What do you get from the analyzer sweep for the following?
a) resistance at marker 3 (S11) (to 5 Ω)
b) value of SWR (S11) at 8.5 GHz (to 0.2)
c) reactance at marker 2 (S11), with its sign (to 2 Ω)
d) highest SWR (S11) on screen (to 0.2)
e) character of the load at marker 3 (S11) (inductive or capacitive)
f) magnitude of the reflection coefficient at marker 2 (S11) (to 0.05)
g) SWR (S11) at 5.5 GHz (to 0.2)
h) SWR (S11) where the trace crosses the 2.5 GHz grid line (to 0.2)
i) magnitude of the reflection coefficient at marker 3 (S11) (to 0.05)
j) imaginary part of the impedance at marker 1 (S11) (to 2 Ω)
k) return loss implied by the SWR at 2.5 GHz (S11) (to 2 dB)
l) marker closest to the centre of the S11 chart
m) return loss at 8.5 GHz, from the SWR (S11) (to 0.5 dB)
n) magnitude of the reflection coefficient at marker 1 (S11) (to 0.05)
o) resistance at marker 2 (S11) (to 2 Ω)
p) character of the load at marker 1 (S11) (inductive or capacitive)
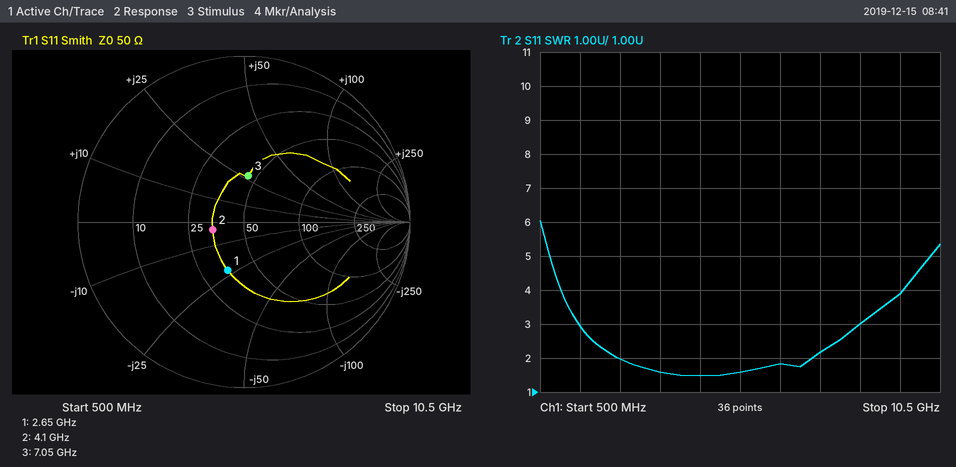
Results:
45 Ω
3.0
-4 Ω
6.0
inductive
0.20
1.6
2.0
0.30
-22 Ω
10 dB
marker 2
6.0 dB
0.30
34 Ω
capacitive
